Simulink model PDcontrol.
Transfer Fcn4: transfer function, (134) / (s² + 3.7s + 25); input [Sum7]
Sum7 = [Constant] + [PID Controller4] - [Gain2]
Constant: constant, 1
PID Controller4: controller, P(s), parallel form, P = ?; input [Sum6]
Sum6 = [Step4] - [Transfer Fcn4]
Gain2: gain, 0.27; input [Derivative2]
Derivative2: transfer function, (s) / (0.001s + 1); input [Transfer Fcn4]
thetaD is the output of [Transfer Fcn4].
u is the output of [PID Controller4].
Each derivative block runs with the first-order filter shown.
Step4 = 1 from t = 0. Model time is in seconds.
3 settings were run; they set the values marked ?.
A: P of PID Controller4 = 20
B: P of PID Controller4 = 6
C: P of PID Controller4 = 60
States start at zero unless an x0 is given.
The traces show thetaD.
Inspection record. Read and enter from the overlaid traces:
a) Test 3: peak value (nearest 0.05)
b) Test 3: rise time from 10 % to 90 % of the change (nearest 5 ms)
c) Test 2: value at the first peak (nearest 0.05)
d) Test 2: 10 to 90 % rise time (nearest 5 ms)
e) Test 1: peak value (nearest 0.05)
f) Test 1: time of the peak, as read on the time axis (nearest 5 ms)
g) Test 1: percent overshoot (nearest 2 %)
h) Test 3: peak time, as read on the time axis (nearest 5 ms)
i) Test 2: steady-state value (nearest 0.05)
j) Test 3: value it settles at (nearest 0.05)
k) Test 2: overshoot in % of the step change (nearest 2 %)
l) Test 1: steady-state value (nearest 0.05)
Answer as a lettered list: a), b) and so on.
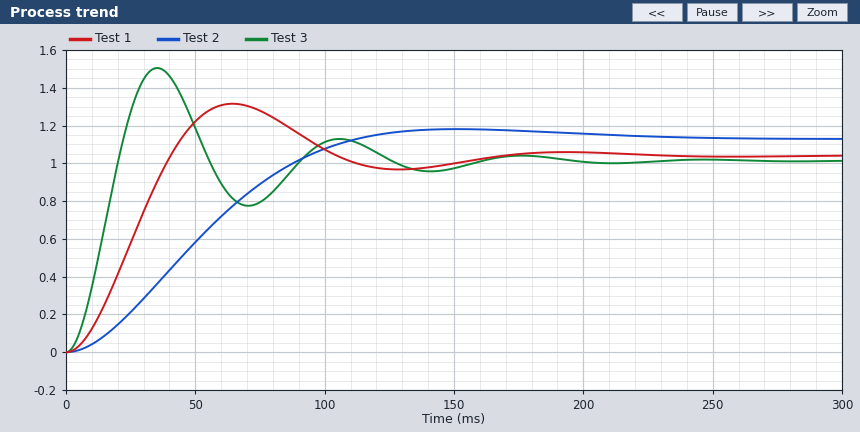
a) 1.50
b) 15 ms
c) 1.20
d) 75 ms
e) 1.30
f) 65 ms
g) 26 %
h) 35 ms
i) 1.15
j) 1.00
k) 4 %
l) 1.05
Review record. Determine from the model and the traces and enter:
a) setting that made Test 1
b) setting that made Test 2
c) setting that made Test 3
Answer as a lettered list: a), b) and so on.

a) A
b) B
c) C
